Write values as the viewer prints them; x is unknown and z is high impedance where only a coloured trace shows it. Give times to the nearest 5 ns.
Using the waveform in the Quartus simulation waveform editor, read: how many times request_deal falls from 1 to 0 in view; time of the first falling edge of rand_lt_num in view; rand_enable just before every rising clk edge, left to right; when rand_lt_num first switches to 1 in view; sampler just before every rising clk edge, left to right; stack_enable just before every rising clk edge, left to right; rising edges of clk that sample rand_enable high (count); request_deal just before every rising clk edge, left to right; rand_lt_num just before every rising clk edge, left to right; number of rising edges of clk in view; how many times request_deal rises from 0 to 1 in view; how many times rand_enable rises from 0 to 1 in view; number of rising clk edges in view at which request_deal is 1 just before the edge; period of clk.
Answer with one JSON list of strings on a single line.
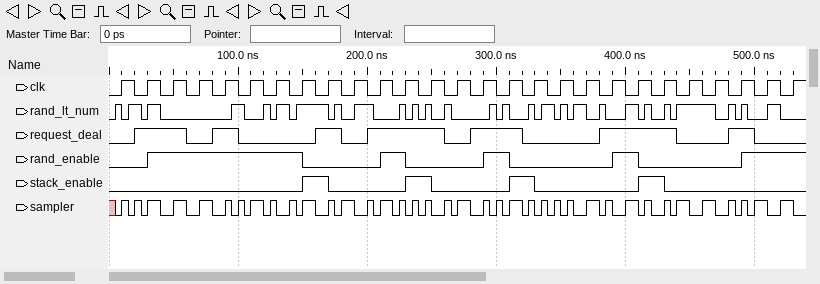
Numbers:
["7", "10 ns", "0 0 1 1 1 1 1 1 0 0 0 1 0 0 0 1 0 0 0 0 1 0 0 0 0 1 1", "5 ns", "0 0 0 0 0 0 1 0 0 1 0 1 1 0 0 0 1 1 0 1 1 0 1 1 0 1 1", "0 0 0 0 0 0 0 0 1 0 0 0 1 0 0 0 1 0 0 0 0 1 0 0 0 0 0", "11", "0 1 1 0 1 0 0 0 1 0 1 1 1 0 1 1 0 0 0 1 1 1 0 0 1 0 0", "1 0 0 0 0 0 0 1 1 0 0 1 1 0 0 1 1 0 1 0 1 0 1 1 0 0 0", "27", "7", "5", "13", "20 ns"]
